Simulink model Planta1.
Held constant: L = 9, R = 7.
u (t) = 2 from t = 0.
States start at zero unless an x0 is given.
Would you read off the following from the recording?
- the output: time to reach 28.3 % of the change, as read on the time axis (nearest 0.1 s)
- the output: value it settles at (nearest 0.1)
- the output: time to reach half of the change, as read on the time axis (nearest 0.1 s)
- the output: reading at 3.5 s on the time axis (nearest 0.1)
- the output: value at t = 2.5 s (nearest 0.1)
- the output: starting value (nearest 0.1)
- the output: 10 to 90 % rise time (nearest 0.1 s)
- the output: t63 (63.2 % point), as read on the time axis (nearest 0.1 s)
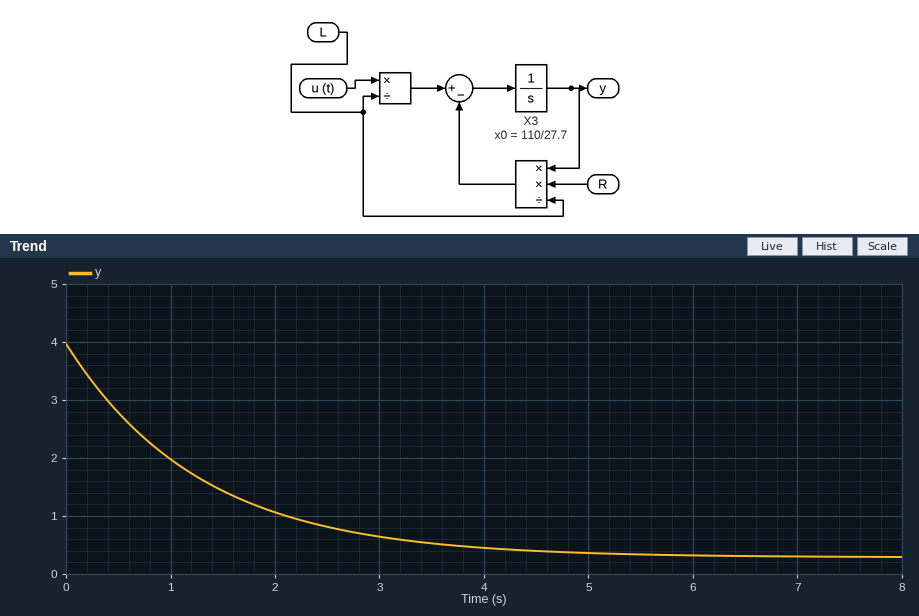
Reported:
0.4 s
0.3
0.9 s
0.5
0.8
4.0
2.8 s
1.3 s
